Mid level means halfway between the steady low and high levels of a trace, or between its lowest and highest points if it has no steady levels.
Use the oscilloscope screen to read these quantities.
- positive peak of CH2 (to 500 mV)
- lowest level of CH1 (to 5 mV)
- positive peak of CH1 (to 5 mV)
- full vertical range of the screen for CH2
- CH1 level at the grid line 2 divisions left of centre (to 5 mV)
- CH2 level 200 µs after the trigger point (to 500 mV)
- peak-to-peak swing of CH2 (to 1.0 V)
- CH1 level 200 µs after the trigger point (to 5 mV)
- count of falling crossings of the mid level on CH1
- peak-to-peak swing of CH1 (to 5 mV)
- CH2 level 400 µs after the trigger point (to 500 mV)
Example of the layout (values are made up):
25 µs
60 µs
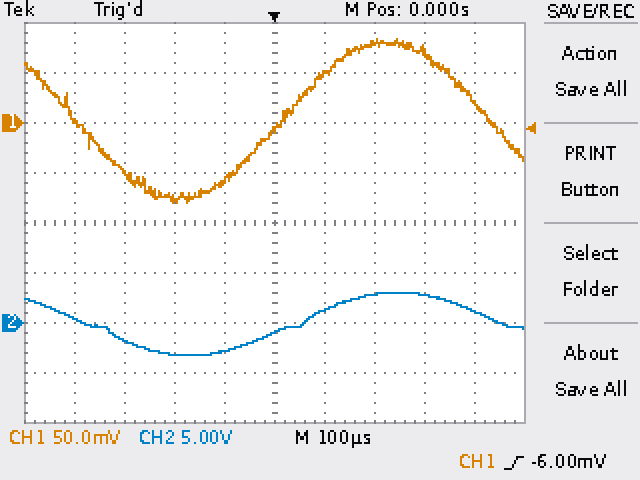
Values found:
3.0 V
-80 mV
85 mV
40 V
-75 mV
3.0 V
6.0 V
80 mV
2
165 mV
1.0 V
